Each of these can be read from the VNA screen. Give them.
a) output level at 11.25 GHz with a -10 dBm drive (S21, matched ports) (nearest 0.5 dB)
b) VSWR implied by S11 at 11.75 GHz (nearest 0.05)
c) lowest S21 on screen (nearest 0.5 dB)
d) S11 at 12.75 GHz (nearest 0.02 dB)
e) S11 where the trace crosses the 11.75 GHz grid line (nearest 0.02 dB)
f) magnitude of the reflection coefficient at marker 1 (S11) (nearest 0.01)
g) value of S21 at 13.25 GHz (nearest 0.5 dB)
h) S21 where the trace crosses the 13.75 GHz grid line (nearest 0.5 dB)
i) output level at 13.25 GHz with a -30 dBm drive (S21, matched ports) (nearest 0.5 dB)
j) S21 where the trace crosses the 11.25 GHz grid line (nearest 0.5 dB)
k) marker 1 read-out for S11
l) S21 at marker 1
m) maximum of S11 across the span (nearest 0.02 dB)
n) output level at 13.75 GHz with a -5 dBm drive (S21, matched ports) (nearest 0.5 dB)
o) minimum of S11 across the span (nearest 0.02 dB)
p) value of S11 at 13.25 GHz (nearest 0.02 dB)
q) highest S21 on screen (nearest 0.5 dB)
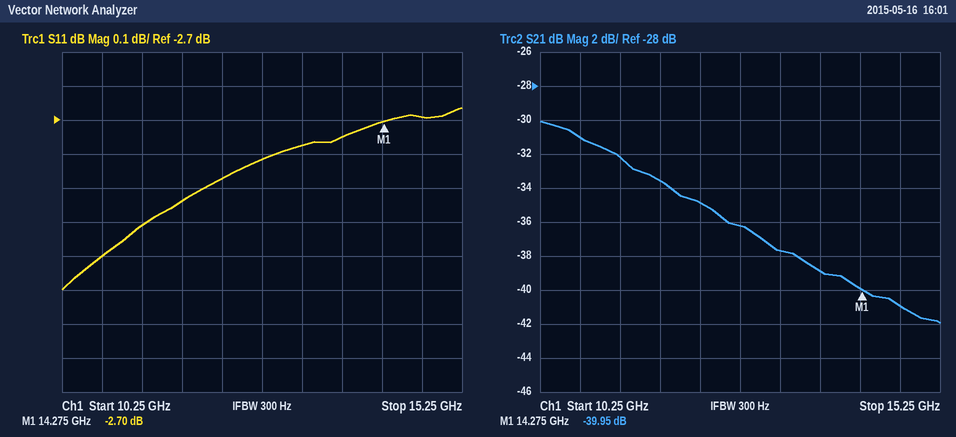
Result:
-42.0 dBm
5.95
-42.0 dB
-2.82 dB
-2.94 dB
0.73
-37.5 dB
-39.0 dB
-67.5 dBm
-32.0 dB
-2.70 dB
-39.95 dB
-2.66 dB
-44.0 dBm
-3.20 dB
-2.78 dB
-30.0 dB
